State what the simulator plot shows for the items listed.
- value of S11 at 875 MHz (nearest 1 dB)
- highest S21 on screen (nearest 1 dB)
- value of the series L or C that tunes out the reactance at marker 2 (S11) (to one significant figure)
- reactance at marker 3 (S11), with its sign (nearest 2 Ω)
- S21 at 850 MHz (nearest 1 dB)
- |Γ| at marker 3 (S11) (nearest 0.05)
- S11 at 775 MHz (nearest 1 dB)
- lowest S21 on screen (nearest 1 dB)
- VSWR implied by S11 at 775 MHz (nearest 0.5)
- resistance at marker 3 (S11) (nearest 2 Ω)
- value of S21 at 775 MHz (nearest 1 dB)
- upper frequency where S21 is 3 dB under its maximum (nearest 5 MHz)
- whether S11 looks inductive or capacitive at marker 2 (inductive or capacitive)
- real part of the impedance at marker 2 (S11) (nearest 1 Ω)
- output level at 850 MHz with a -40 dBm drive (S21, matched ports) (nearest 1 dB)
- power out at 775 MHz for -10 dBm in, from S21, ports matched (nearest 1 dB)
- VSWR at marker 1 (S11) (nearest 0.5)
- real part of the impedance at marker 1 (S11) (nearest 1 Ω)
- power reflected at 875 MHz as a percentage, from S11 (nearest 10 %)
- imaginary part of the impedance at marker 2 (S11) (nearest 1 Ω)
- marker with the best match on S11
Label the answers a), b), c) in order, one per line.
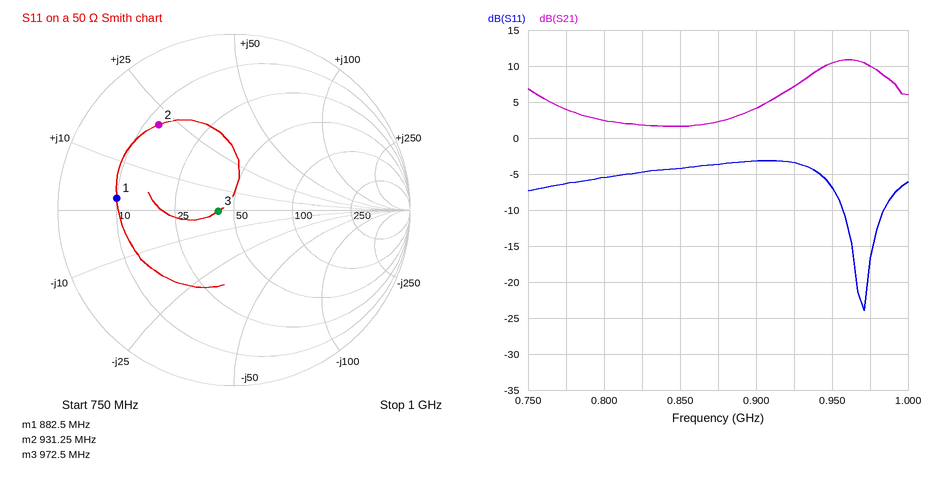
a) -4 dB
b) 11 dB
c) 8 pF
d) 0 Ω
e) 2 dB
f) 0.10
g) -6 dB
h) 2 dB
i) 3.0
j) 42 Ω
k) 4 dB
l) 990 MHz
m) inductive
n) 13 Ω
o) -38 dBm
p) -6 dBm
q) 5.0
r) 10 Ω
s) 40 %
t) +21 Ω
u) marker 3
